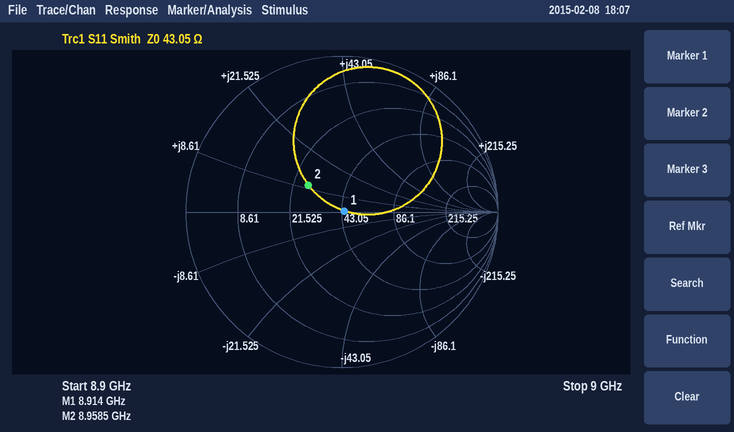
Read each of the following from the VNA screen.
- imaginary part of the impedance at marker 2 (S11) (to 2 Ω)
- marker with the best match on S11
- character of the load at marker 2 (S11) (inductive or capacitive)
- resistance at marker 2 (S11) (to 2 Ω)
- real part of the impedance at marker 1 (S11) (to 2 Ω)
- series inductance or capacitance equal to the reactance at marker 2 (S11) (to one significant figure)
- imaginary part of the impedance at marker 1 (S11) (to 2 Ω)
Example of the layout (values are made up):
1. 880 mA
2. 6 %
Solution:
1. +10 Ω
2. marker 1
3. inductive
4. 26 Ω
5. 44 Ω
6. 200 pH
7. 0 Ω
